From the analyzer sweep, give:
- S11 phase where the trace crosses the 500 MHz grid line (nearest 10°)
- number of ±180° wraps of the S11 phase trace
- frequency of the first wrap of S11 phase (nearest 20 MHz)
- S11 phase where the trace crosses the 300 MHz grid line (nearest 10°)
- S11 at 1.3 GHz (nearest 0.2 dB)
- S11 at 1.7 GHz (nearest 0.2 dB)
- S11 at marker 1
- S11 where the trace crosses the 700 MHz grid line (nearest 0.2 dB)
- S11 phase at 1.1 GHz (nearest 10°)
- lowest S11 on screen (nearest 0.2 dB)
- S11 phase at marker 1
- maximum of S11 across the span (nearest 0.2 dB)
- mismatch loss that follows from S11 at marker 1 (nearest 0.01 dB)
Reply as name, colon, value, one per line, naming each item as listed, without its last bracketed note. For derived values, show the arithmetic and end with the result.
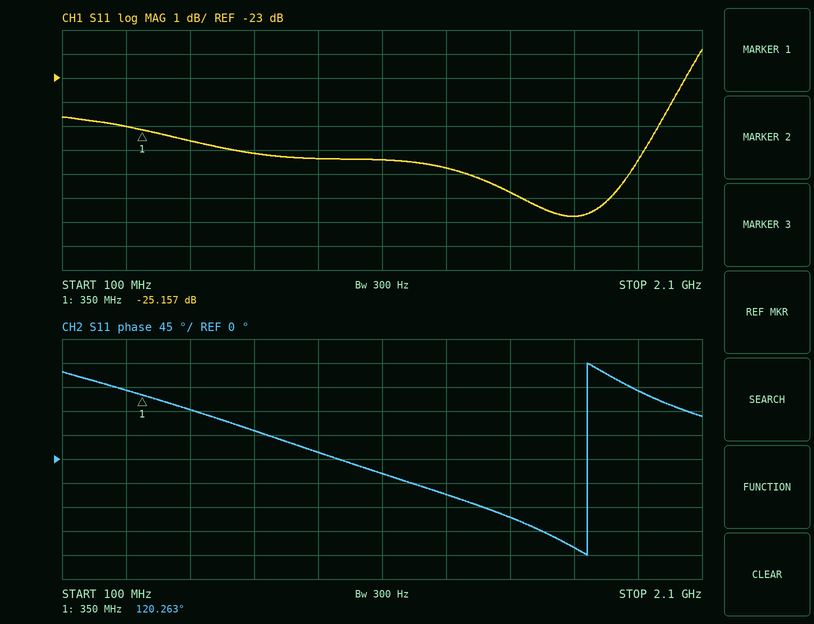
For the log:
S11 phase where the trace crosses the 500 MHz grid line: 90°
number of ±180° wraps of the S11 phase trace: 1
frequency of the first wrap of S11 phase: 1.74 GHz
S11 phase where the trace crosses the 300 MHz grid line: 130°
S11 at 1.3 GHz: -26.8 dB
S11 at 1.7 GHz: -28.8 dB
S11 at marker 1: -25.157 dB
S11 where the trace crosses the 700 MHz grid line: -26.2 dB
S11 phase at 1.1 GHz: -30°
lowest S11 on screen: -28.8 dB
S11 phase at marker 1: 120.263°
maximum of S11 across the span: -21.8 dB
mismatch loss that follows from S11 at marker 1: −10 log10(1 − 10^(-25.157/10)) ≈ 0.01 dB
